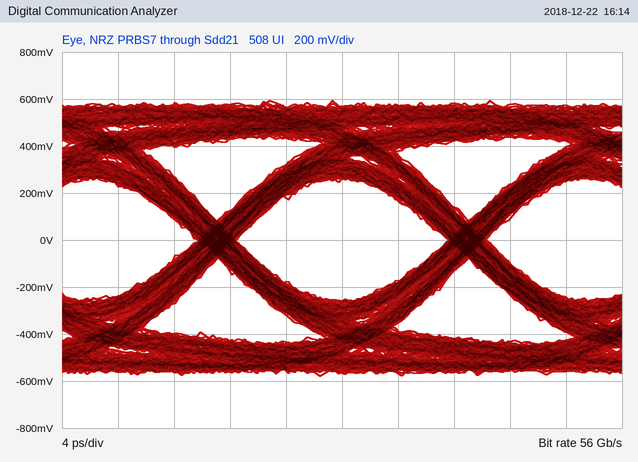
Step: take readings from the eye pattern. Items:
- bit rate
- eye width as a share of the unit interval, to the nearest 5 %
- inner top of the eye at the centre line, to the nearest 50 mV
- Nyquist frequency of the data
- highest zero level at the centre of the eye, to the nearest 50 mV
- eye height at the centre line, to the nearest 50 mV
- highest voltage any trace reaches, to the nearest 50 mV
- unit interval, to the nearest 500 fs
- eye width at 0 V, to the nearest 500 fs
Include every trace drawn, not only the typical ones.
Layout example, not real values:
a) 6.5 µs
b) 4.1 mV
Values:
a) 56 Gb/s
b) 85 %
c) 250 mV
d) 28 GHz
e) -250 mV
f) 500 mV
g) 600 mV
h) 18.0 ps
i) 15.0 ps
